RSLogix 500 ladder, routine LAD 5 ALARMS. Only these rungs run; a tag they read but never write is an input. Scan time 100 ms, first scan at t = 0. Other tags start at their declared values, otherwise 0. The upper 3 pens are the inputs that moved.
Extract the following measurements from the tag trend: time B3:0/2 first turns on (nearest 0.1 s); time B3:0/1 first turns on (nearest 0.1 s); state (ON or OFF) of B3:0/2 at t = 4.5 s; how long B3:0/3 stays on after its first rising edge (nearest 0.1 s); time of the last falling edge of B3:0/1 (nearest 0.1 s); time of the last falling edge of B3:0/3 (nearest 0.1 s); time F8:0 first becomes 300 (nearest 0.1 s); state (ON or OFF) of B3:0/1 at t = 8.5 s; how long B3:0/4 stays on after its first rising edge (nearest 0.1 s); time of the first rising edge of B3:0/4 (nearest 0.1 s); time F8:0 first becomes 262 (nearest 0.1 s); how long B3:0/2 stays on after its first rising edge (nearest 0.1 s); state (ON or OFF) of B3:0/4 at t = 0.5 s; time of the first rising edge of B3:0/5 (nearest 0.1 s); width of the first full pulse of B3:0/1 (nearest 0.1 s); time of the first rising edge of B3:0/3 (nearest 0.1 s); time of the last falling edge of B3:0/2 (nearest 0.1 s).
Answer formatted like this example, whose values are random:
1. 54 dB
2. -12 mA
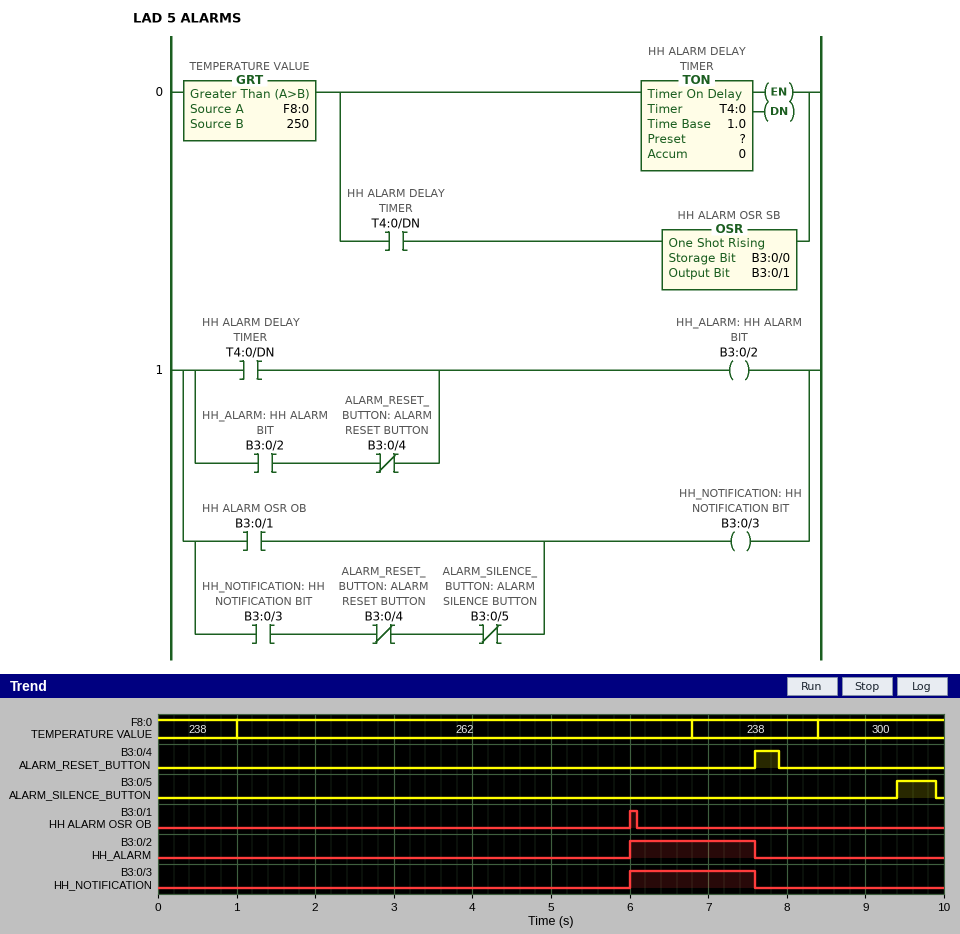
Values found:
1. 6.0 s
2. 6.0 s
3. OFF
4. 1.6 s
5. 6.1 s
6. 7.6 s
7. 8.4 s
8. OFF
9. 0.3 s
10. 7.6 s
11. 1.0 s
12. 1.6 s
13. OFF
14. 9.4 s
15. 0.1 s
16. 6.0 s
17. 7.6 s
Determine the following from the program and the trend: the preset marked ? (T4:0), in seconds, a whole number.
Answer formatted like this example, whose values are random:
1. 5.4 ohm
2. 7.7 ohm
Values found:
1. 5 s
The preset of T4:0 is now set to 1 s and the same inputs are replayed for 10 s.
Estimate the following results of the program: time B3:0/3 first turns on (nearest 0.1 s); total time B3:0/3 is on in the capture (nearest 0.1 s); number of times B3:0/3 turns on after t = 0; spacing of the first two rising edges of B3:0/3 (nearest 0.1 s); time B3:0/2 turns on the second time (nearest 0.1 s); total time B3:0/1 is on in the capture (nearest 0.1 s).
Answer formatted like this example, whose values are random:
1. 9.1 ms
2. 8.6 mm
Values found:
1. 2.0 s
2. 5.7 s
3. 2
4. 7.4 s
5. 9.4 s
6. 0.2 s
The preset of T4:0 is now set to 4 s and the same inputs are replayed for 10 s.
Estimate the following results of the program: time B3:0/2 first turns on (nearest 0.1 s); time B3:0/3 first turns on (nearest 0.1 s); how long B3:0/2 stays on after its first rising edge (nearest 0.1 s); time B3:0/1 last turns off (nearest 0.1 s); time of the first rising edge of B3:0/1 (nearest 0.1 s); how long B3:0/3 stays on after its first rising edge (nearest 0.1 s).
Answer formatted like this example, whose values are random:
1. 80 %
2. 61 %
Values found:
1. 5.0 s
2. 5.0 s
3. 2.6 s
4. 5.1 s
5. 5.0 s
6. 2.6 s
